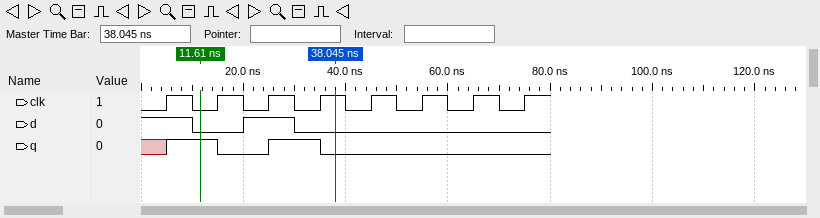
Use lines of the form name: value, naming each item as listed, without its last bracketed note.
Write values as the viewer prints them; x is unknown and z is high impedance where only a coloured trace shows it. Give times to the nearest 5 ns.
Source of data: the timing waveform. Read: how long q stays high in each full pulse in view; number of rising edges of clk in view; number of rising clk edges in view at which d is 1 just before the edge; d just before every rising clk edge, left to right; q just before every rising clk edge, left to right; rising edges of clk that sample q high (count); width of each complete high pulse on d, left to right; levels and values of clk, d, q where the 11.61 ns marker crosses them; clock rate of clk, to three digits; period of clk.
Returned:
how long q stays high in each full pulse in view: 10 ns
number of rising edges of clk in view: 8
number of rising clk edges in view at which d is 1 just before the edge: 2
d just before every rising clk edge, left to right: 1 0 1 0 0 0 0 0
q just before every rising clk edge, left to right: x 1 0 1 0 0 0 0
rising edges of clk that sample q high: 2
width of each complete high pulse on d, left to right: 10 ns
levels and values of clk, d, q where the 11.61 ns marker crosses them: clk=0, d=0, q=1
clock rate of clk, to three digits: 100 MHz
period of clk: 10 ns
